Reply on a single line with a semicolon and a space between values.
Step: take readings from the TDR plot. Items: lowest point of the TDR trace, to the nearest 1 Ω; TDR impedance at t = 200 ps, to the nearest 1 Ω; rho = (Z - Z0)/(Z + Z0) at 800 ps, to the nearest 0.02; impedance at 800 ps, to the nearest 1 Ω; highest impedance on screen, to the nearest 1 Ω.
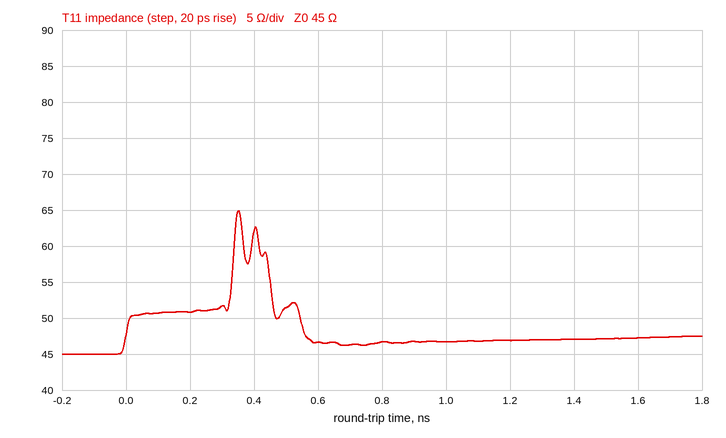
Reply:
45 Ω; 51 Ω; +0.02; 47 Ω; 65 Ω
